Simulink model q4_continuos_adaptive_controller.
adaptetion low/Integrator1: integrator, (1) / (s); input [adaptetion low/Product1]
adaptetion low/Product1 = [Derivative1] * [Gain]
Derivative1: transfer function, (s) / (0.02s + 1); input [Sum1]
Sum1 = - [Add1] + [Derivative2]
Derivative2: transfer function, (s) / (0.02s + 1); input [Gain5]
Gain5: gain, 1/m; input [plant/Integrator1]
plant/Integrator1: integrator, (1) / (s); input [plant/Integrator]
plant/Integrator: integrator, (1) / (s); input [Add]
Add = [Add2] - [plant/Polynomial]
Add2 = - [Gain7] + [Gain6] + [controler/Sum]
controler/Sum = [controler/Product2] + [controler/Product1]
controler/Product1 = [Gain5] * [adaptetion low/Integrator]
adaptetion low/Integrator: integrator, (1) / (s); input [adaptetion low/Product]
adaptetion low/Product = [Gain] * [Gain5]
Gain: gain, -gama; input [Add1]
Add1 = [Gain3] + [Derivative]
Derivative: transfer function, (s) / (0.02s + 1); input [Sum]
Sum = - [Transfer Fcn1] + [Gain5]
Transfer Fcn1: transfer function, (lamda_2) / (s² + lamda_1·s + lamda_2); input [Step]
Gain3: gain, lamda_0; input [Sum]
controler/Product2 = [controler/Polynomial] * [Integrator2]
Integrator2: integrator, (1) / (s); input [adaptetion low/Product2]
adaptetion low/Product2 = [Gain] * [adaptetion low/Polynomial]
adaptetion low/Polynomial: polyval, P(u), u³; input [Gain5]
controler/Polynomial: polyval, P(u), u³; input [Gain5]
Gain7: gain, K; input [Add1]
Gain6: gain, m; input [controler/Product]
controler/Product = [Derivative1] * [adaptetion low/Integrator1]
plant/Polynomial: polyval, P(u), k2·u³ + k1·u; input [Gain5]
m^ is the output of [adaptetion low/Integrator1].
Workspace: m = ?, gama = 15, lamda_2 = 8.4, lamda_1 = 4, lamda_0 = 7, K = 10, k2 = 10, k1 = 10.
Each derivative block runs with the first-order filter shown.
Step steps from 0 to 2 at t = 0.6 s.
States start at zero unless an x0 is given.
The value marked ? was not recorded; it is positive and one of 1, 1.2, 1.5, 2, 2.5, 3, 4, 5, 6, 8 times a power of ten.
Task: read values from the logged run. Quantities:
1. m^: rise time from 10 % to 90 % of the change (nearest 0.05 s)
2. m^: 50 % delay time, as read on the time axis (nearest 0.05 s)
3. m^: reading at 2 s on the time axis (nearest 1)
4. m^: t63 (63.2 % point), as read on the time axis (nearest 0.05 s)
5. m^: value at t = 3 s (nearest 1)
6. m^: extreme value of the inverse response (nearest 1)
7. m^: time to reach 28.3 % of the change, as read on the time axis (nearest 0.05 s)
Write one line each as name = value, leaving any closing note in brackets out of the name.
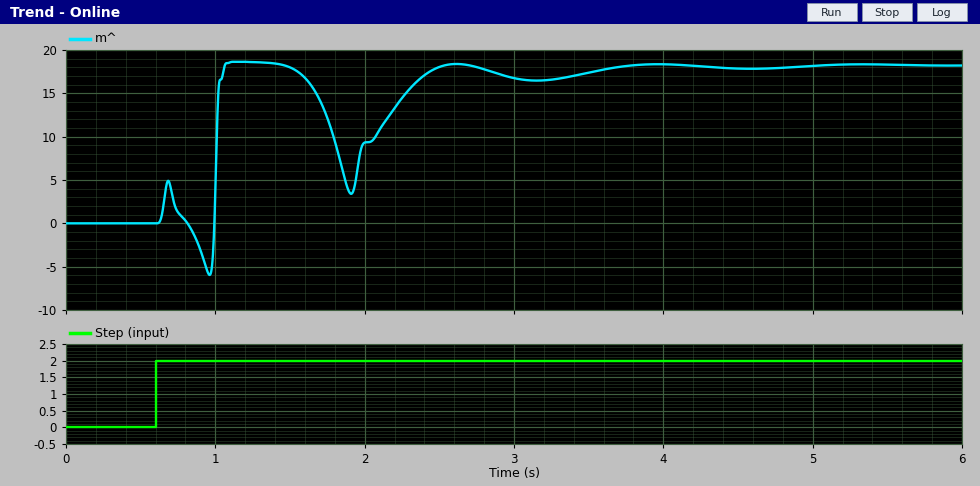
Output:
m^: rise time from 10 % to 90 % of the change = 0.40 s
m^: 50 % delay time, as read on the time axis = 1.00 s
m^: reading at 2 s on the time axis = 9
m^: t63 (63.2 % point), as read on the time axis = 1.00 s
m^: value at t = 3 s = 17
m^: extreme value of the inverse response = -6
m^: time to reach 28.3 % of the change, as read on the time axis = 1.00 s
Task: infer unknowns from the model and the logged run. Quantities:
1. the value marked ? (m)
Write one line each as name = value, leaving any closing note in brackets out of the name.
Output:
the value marked ? = 10
